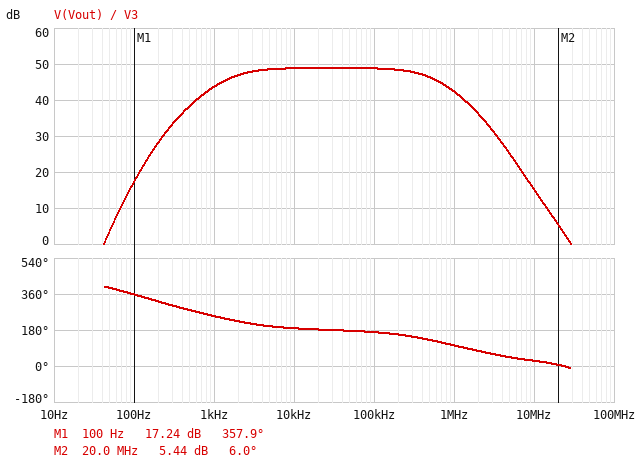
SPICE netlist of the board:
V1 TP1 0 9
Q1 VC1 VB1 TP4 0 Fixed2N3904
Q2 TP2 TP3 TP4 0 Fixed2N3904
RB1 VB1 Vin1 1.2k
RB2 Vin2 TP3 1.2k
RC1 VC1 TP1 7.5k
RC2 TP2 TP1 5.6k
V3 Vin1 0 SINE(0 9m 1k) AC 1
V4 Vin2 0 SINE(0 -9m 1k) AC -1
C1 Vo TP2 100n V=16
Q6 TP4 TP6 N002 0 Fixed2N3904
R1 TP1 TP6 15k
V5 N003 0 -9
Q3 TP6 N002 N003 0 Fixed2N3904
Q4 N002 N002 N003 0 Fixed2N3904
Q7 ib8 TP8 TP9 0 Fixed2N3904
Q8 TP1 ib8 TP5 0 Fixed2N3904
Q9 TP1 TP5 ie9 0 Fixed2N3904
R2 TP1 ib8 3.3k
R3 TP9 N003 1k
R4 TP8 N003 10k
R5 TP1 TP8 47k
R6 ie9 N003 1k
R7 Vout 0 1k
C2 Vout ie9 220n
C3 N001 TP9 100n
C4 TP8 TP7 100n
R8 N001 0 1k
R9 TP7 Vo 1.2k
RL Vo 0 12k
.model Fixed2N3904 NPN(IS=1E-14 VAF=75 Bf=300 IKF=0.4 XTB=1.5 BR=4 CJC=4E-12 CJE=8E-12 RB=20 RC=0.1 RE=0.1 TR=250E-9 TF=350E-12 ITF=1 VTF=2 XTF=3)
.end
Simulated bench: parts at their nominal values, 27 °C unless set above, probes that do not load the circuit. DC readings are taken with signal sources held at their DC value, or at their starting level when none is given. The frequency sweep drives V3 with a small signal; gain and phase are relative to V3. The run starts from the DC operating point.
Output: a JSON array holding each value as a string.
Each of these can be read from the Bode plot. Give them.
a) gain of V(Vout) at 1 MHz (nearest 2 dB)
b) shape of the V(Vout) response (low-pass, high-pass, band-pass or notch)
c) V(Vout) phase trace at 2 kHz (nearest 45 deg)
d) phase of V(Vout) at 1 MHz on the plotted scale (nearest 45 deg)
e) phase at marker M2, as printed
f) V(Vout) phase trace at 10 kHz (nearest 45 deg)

["42 dB", "band-pass", "225 deg", "90 deg", "6.0 deg", "180 deg"]
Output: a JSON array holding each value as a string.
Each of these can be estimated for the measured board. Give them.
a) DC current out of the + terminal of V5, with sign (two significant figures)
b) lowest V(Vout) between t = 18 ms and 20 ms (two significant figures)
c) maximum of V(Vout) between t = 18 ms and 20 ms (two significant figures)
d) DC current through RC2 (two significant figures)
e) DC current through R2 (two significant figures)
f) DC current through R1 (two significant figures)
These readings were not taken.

["-14 mA", "-1.4 V", "1.4 V", "550 µA", "2.4 mA", "1.1 mA"]
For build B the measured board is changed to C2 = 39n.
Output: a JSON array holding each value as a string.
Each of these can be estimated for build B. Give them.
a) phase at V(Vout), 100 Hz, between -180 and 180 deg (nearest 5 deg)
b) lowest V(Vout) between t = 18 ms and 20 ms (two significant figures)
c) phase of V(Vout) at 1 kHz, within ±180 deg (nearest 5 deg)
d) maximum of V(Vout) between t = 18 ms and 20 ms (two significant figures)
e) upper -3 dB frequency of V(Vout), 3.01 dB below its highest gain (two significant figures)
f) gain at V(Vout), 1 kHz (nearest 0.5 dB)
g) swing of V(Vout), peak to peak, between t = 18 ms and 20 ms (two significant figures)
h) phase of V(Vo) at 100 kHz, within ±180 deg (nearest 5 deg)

["5 deg", "-400 mV", "-70 deg", "400 mV", "560 kHz", "33.0 dB", "800 mV", "-10 deg"]
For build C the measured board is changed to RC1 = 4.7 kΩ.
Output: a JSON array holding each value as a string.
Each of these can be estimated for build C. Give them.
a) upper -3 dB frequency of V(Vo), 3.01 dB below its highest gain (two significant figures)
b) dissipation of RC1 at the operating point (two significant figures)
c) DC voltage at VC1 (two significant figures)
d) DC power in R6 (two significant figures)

["740 kHz", "1.4 mW", "6.4 V", "77 mW"]
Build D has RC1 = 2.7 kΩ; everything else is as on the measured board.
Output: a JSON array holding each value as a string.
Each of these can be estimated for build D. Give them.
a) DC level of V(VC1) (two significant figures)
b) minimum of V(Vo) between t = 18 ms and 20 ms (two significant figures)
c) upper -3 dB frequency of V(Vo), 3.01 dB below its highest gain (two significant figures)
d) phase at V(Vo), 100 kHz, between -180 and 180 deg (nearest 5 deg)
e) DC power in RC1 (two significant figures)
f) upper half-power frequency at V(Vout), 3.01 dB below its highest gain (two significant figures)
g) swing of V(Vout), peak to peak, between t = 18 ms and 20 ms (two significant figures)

["7.5 V", "-450 mV", "940 kHz", "-5 deg", "830 µW", "920 kHz", "2.8 V"]
